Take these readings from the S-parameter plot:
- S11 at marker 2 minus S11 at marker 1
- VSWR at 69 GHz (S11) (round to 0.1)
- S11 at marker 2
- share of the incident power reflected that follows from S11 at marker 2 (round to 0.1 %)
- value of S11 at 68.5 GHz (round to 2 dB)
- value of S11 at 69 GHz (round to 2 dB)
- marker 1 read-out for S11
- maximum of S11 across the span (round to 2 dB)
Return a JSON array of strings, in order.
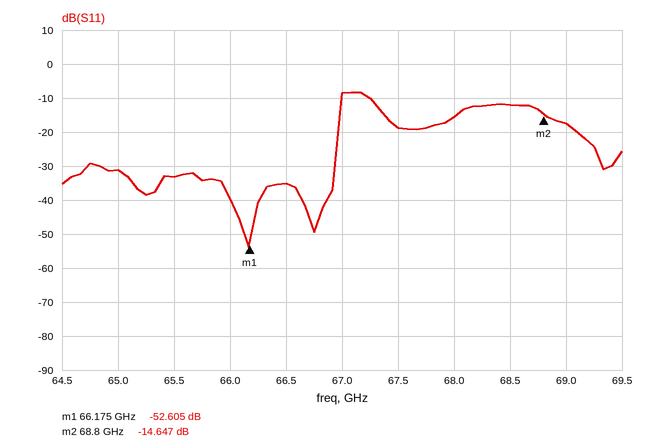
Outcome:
["37.958 dB", "1.3", "-14.647 dB", "3.4 %", "-12 dB", "-18 dB", "-52.605 dB", "-8 dB"]
